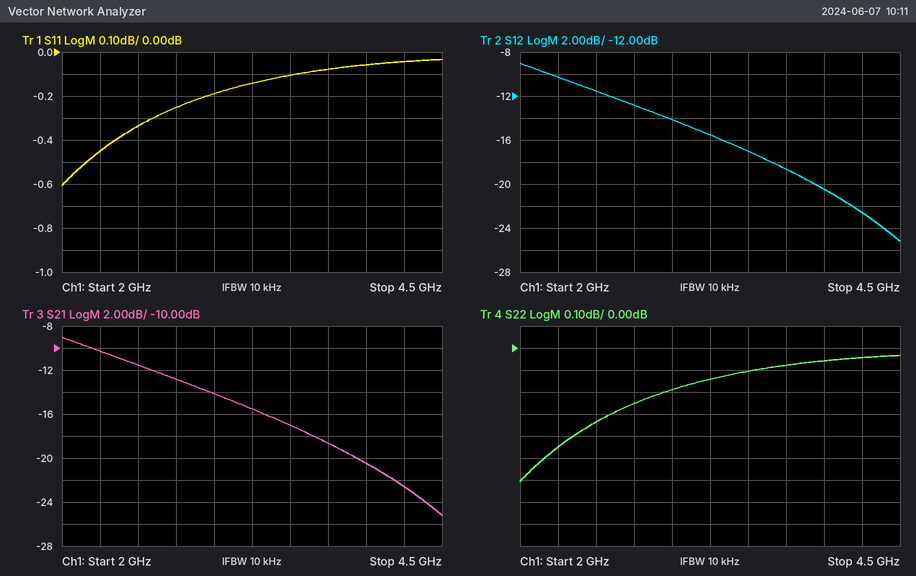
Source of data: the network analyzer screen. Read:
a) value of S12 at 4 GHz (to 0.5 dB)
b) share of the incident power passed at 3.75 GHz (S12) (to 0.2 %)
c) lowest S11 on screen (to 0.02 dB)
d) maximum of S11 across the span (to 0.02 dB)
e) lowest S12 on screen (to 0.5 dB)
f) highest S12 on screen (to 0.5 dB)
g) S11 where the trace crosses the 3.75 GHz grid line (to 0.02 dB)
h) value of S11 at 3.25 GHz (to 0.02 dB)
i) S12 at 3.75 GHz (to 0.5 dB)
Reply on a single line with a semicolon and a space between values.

-20.5 dB; 1.4 %; -0.60 dB; -0.04 dB; -25.0 dB; -9.0 dB; -0.08 dB; -0.14 dB; -18.5 dB
